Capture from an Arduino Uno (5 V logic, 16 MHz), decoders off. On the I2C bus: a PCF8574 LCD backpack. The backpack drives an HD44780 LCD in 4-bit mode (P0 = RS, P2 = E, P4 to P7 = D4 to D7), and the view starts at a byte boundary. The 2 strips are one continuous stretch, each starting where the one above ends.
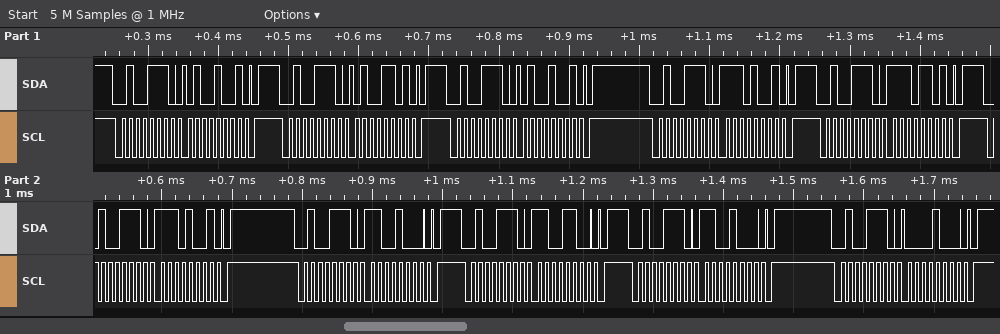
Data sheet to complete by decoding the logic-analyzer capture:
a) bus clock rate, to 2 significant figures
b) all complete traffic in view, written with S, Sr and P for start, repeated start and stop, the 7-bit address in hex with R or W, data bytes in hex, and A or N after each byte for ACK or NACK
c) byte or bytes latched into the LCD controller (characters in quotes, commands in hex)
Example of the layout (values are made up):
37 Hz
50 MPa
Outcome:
100 kHz
S 27W A 49 A P S 27W A 4D A P S 27W A 49 A P S 27W A E9 A P S 27W A ED A P S 27W A E9 A P S 27W A C8 A P S 27W A CC A P S 27W A C8 A P S 27W A 08 A P
'N'
